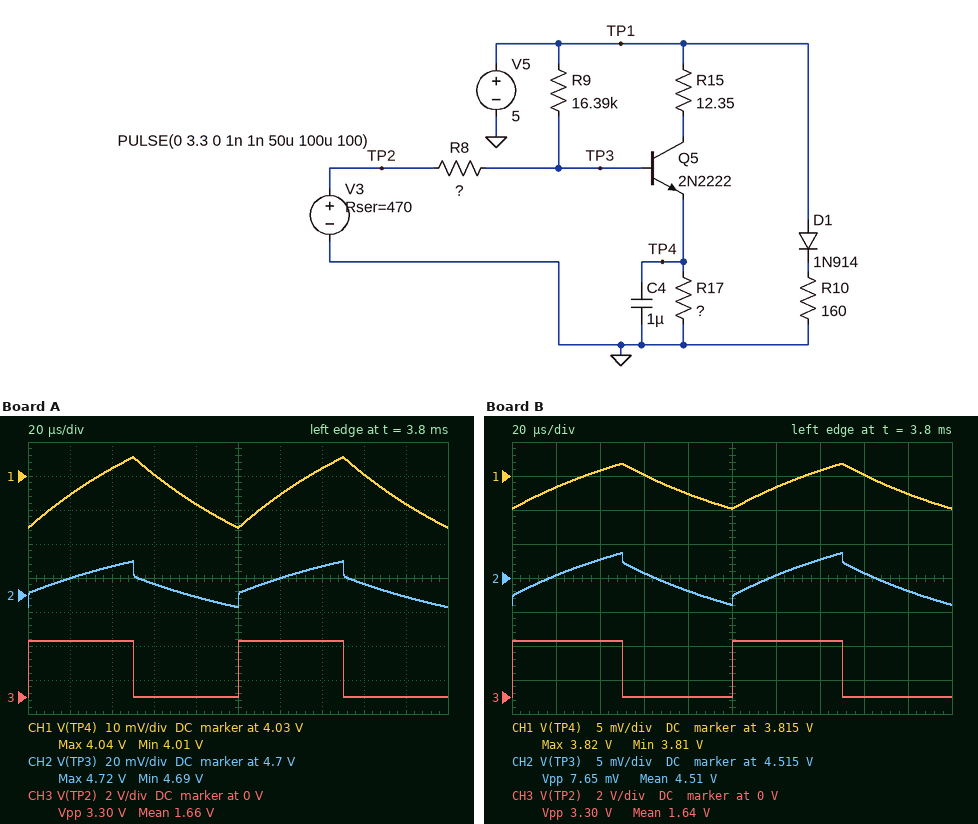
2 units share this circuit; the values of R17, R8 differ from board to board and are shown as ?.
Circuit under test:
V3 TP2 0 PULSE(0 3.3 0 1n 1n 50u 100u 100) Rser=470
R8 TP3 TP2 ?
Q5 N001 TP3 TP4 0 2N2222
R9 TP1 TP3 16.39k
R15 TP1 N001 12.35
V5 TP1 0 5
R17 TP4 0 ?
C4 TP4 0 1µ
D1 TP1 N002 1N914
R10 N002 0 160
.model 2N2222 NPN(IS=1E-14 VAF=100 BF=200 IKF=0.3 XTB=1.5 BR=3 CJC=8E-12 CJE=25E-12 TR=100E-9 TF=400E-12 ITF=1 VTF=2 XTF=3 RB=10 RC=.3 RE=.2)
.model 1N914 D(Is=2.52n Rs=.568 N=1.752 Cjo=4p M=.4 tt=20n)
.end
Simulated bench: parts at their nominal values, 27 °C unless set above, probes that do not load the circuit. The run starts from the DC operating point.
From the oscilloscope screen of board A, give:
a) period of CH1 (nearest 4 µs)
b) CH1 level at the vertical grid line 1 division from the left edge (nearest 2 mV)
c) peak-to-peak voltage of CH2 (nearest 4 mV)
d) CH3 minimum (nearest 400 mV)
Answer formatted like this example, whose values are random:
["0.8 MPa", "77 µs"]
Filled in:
["100 µs", "4.024 V", "28 mV", "0 V"]
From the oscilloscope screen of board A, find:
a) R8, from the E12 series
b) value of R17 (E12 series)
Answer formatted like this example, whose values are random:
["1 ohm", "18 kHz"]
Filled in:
["680 kΩ", "1.5 kΩ"]
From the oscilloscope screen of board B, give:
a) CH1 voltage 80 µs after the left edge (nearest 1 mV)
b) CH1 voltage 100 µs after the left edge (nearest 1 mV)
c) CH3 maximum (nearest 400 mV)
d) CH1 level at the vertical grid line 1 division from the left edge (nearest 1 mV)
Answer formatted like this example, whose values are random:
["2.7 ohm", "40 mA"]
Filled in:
["3.812 V", "3.810 V", "3.2 V", "3.813 V"]
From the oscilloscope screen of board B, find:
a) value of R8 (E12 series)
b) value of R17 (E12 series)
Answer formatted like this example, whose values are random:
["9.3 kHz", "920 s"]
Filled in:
["2.2 MΩ", "680 Ω"]
